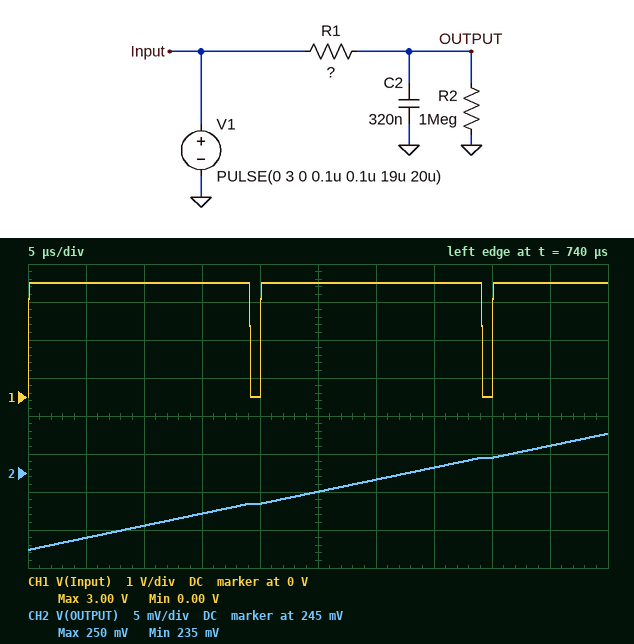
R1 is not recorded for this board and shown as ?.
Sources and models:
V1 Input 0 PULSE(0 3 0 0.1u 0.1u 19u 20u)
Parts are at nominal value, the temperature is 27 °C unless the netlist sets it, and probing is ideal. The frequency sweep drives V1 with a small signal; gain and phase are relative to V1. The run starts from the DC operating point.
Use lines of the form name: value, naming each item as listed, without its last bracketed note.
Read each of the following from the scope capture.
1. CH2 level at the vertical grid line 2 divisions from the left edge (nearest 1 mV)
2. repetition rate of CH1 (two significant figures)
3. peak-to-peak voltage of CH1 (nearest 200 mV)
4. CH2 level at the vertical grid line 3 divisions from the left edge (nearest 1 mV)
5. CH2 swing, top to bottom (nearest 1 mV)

CH2 level at the vertical grid line 2 divisions from the left edge: 238 mV
repetition rate of CH1: 50 kHz
peak-to-peak voltage of CH1: 3.0 V
CH2 level at the vertical grid line 3 divisions from the left edge: 240 mV
CH2 swing, top to bottom: 15 mV
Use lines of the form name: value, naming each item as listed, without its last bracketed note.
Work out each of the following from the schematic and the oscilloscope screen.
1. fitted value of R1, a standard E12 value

fitted value of R1, a standard E12 value: 27 kΩ
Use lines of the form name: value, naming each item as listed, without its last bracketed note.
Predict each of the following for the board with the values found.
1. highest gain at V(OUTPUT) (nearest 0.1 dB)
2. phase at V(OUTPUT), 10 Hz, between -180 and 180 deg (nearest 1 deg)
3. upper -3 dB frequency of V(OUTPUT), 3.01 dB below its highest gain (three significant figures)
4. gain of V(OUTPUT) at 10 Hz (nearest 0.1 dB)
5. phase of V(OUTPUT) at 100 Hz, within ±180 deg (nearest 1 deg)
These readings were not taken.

highest gain at V(OUTPUT): -0.2 dB
phase at V(OUTPUT), 10 Hz, between -180 and 180 deg: -28 deg
upper -3 dB frequency of V(OUTPUT), 3.01 dB below its highest gain: 18.9 Hz
gain of V(OUTPUT) at 10 Hz: -1.3 dB
phase of V(OUTPUT) at 100 Hz, within ±180 deg: -79 deg
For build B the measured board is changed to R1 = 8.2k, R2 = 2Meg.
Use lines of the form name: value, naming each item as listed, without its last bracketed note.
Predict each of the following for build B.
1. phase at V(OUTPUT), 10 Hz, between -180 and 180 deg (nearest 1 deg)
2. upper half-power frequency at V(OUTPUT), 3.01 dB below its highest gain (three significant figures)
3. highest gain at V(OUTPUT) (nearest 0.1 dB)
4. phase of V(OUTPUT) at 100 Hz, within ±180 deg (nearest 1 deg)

phase at V(OUTPUT), 10 Hz, between -180 and 180 deg: -9 deg
upper half-power frequency at V(OUTPUT), 3.01 dB below its highest gain: 60.9 Hz
highest gain at V(OUTPUT): 0 dB
phase of V(OUTPUT) at 100 Hz, within ±180 deg: -59 deg
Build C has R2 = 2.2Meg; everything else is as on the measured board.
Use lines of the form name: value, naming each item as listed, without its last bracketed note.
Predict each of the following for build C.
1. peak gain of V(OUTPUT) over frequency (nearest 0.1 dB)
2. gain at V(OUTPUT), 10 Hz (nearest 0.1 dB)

peak gain of V(OUTPUT) over frequency: -0.1 dB
gain at V(OUTPUT), 10 Hz: -1.2 dB
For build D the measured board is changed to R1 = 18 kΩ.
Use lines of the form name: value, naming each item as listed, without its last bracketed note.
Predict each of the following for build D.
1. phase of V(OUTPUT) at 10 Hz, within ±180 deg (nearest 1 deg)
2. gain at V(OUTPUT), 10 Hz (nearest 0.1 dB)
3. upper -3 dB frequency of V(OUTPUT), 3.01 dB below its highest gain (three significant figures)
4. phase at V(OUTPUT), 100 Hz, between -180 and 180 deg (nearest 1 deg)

phase of V(OUTPUT) at 10 Hz, within ±180 deg: -20 deg
gain at V(OUTPUT), 10 Hz: -0.7 dB
upper -3 dB frequency of V(OUTPUT), 3.01 dB below its highest gain: 28.1 Hz
phase at V(OUTPUT), 100 Hz, between -180 and 180 deg: -74 deg
